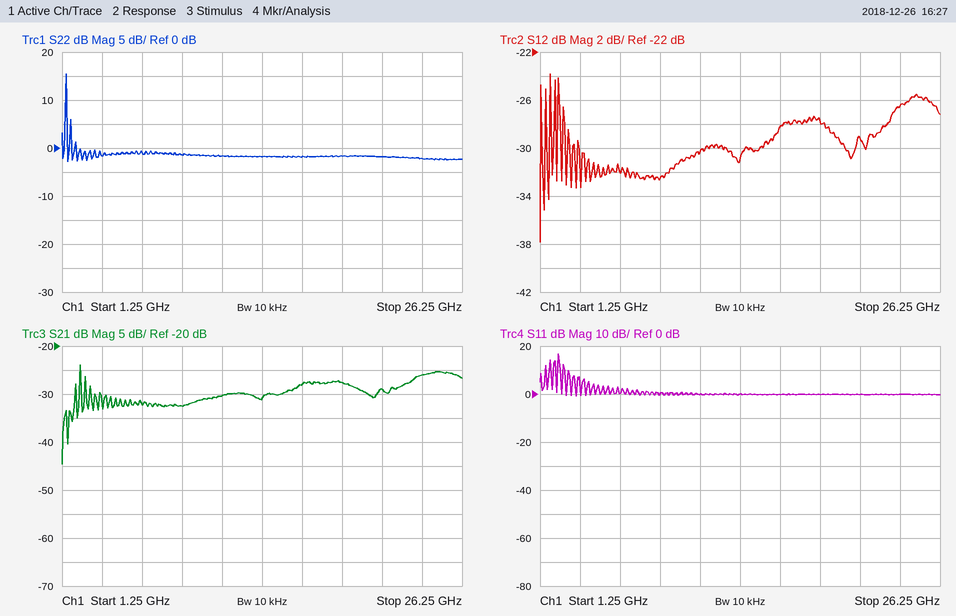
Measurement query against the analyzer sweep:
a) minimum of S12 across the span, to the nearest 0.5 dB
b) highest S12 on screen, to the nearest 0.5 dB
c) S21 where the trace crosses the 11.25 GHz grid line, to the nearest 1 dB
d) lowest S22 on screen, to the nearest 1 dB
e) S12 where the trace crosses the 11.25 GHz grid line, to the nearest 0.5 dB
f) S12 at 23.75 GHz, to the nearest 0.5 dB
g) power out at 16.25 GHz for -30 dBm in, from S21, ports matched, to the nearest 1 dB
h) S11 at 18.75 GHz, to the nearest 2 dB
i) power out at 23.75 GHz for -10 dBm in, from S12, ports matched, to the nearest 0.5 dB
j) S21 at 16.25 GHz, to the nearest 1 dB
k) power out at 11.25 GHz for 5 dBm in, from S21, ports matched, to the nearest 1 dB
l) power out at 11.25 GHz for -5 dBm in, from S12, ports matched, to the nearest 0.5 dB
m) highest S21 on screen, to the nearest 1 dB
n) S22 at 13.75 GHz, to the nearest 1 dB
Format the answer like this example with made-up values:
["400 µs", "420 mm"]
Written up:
["-38.0 dB", "-24.0 dB", "-30 dB", "-3 dB", "-30.5 dB", "-26.5 dB", "-58 dBm", "0 dB", "-36.5 dBm", "-28 dB", "-25 dBm", "-35.5 dBm", "-24 dB", "-2 dB"]
